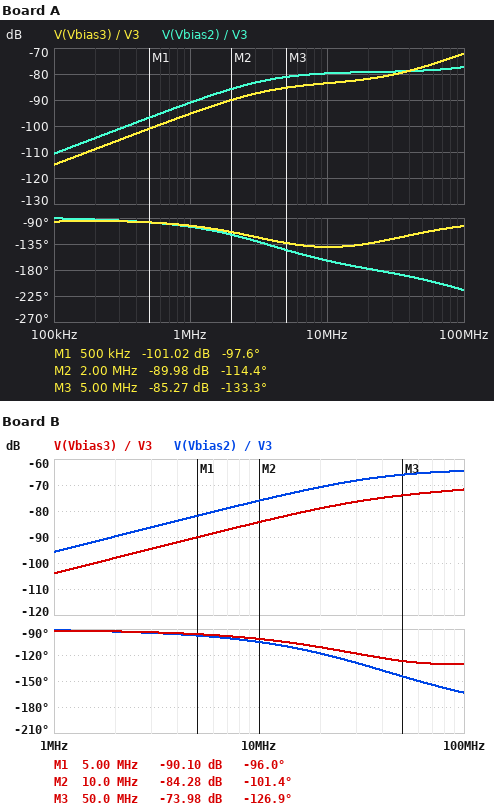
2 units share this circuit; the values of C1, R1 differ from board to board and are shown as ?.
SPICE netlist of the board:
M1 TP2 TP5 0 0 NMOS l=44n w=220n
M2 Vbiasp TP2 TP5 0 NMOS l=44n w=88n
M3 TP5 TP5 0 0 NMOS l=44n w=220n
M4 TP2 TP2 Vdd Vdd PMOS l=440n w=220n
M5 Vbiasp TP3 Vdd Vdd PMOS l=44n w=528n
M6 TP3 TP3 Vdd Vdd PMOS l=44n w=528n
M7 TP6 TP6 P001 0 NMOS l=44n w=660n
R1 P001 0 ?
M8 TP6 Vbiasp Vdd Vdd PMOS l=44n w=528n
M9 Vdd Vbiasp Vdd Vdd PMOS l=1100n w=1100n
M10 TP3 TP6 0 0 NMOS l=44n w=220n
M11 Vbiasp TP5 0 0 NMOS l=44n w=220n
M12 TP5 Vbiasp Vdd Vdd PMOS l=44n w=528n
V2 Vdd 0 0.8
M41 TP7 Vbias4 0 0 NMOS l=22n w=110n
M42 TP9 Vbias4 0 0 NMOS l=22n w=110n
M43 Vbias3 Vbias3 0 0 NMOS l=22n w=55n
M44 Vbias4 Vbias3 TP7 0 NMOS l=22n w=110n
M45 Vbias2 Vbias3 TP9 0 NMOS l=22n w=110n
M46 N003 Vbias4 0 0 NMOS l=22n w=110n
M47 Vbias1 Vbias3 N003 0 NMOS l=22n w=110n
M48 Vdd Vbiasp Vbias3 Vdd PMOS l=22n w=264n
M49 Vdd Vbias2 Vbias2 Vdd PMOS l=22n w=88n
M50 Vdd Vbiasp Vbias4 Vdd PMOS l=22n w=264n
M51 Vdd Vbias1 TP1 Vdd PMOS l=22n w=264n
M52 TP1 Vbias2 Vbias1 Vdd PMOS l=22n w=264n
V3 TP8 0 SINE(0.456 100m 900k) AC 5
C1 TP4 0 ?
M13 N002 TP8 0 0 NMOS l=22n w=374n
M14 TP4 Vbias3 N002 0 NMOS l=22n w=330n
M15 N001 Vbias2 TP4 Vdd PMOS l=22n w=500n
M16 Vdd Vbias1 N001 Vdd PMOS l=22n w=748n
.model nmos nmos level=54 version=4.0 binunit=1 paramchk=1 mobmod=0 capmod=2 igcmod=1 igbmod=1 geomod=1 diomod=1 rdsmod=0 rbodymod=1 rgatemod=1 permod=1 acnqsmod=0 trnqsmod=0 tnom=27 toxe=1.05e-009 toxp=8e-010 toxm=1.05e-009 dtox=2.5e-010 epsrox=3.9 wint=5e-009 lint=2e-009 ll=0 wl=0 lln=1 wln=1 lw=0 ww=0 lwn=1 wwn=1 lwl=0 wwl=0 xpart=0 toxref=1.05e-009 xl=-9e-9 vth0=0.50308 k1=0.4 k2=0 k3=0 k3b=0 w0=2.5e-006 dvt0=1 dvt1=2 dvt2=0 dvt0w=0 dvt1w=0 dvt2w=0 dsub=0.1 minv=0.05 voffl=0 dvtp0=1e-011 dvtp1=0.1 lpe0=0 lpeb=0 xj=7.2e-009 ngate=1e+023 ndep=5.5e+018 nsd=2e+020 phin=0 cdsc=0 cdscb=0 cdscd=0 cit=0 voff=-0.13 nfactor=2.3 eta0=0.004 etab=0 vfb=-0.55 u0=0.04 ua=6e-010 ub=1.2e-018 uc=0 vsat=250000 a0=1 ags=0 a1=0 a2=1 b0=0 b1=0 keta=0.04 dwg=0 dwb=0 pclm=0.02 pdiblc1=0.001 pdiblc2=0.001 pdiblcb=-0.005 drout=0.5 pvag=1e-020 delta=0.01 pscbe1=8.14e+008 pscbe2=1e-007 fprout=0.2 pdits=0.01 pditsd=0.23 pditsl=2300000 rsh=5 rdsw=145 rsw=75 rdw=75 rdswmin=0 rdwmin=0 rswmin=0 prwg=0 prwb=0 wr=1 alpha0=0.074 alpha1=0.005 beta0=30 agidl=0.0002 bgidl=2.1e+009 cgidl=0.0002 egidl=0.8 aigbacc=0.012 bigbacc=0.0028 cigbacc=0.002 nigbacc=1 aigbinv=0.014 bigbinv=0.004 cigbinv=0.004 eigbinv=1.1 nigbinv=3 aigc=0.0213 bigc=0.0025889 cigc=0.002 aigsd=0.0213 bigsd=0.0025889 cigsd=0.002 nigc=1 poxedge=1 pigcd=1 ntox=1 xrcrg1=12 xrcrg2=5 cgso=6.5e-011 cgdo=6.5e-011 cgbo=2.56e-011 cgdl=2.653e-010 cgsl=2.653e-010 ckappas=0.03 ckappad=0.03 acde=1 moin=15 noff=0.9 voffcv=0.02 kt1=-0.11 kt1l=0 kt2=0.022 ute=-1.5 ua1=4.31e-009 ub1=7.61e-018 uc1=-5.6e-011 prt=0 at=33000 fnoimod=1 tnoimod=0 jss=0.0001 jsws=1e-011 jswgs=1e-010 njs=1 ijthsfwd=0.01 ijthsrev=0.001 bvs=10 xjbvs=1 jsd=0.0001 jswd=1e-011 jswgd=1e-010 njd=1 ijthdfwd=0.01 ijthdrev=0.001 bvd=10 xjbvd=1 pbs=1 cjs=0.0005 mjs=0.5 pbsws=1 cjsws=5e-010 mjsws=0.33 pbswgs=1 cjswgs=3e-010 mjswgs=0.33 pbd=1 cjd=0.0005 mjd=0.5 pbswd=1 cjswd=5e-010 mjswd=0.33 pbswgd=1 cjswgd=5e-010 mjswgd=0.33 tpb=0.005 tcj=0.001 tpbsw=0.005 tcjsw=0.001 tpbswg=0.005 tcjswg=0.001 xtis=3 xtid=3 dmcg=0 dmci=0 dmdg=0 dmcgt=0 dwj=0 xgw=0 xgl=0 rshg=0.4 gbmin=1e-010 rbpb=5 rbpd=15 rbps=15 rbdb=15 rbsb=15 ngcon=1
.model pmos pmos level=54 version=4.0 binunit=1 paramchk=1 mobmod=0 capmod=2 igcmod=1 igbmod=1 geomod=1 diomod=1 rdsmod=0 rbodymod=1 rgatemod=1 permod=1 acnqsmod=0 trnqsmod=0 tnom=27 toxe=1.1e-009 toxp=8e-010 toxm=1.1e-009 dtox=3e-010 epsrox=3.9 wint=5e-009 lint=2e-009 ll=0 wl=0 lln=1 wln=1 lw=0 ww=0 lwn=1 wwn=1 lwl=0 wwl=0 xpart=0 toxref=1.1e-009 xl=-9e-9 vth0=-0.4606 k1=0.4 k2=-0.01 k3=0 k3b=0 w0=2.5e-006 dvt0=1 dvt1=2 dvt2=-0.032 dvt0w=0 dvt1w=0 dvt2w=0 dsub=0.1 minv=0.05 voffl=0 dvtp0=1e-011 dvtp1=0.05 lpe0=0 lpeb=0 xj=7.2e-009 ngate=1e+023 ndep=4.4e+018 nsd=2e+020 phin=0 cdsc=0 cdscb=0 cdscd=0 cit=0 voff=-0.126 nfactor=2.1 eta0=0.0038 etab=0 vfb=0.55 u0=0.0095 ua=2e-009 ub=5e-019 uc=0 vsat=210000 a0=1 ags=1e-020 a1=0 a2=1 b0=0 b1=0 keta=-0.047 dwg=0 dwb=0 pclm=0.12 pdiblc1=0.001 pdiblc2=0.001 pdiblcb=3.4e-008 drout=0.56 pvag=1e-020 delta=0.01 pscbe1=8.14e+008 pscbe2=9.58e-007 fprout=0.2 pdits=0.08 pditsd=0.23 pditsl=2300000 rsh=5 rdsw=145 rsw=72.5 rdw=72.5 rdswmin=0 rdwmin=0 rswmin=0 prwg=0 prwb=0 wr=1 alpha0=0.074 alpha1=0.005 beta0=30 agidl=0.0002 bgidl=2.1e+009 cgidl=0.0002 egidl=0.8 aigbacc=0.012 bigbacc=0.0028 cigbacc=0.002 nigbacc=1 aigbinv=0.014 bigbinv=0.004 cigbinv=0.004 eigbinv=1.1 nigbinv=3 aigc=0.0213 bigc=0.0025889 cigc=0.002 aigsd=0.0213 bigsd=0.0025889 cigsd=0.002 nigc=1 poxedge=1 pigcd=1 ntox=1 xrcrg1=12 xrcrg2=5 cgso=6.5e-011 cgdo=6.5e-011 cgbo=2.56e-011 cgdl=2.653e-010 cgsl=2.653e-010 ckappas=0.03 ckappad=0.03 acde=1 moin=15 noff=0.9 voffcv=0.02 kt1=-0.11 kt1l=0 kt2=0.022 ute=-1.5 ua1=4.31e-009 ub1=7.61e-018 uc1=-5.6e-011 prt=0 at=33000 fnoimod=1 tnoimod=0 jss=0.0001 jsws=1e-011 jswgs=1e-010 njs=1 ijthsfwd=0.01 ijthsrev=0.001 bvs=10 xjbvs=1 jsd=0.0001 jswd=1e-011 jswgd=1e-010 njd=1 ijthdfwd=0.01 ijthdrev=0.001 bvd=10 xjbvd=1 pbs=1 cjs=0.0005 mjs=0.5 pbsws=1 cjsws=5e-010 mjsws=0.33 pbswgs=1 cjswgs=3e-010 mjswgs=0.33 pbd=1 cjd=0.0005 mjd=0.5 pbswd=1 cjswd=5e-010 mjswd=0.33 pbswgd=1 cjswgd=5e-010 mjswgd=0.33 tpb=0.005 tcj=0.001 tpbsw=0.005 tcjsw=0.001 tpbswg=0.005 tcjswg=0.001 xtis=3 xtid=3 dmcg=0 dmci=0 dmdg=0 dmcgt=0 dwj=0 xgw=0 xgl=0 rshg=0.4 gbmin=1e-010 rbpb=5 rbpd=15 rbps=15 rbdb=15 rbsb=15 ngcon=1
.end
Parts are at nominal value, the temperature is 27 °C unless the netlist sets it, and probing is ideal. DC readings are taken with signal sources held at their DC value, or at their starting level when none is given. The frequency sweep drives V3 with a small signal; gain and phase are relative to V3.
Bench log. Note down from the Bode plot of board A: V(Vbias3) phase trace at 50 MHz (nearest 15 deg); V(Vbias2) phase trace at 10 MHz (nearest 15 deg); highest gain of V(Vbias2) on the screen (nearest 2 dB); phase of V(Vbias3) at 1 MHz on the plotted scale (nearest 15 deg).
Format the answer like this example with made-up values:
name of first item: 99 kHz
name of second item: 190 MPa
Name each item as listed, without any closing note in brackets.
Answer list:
V(Vbias3) phase trace at 50 MHz: -120 deg
V(Vbias2) phase trace at 10 MHz: -165 deg
highest gain of V(Vbias2) on the screen: -78 dB
phase of V(Vbias3) at 1 MHz on the plotted scale: -105 deg
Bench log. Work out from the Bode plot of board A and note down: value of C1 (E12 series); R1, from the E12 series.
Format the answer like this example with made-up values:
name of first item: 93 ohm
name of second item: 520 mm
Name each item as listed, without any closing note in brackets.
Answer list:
value of C1: 2.7 pF
R1, from the E12 series: 12 kΩ
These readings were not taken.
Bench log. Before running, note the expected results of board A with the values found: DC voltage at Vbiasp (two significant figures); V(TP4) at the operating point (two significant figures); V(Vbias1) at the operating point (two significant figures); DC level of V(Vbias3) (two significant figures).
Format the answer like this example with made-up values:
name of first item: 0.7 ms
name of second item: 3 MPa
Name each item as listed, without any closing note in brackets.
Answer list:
DC voltage at Vbiasp: 310 mV
V(TP4) at the operating point: 500 mV
V(Vbias1) at the operating point: 270 mV
DC level of V(Vbias3): 550 mV
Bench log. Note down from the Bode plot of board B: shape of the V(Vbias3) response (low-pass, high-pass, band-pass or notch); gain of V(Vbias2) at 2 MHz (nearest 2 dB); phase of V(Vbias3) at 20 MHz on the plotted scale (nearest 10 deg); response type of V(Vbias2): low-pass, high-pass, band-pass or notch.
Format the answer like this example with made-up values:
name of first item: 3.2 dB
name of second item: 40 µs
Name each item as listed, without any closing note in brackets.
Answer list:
shape of the V(Vbias3) response: high-pass
gain of V(Vbias2) at 2 MHz: -90 dB
phase of V(Vbias3) at 20 MHz on the plotted scale: -110 deg
response type of V(Vbias2): low-pass, high-pass, band-pass or notch: high-pass
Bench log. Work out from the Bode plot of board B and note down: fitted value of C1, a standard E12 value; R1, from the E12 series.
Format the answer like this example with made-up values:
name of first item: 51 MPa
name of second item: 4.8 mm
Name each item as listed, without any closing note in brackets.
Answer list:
fitted value of C1, a standard E12 value: 560 fF
R1, from the E12 series: 1.8 kΩ
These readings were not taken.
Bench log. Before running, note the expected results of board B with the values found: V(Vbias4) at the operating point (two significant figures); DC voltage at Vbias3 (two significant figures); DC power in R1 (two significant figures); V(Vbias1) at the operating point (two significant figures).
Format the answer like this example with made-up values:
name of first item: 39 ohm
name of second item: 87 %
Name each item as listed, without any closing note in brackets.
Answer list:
V(Vbias4) at the operating point: 690 mV
DC voltage at Vbias3: 680 mV
DC power in R1: 1.9 µW
V(Vbias1) at the operating point: 210 mV
